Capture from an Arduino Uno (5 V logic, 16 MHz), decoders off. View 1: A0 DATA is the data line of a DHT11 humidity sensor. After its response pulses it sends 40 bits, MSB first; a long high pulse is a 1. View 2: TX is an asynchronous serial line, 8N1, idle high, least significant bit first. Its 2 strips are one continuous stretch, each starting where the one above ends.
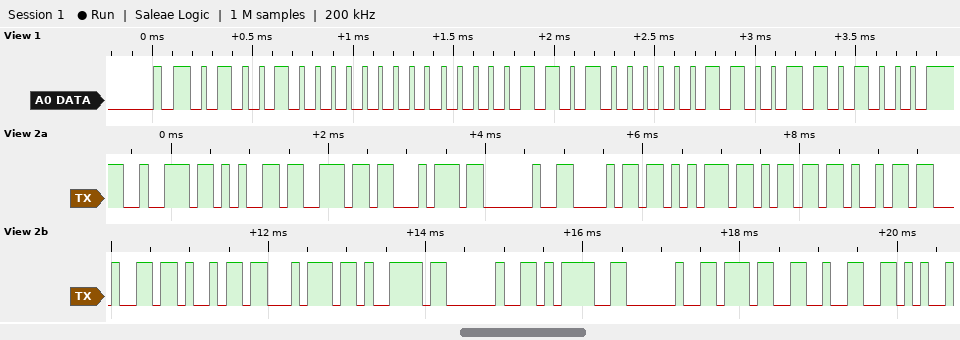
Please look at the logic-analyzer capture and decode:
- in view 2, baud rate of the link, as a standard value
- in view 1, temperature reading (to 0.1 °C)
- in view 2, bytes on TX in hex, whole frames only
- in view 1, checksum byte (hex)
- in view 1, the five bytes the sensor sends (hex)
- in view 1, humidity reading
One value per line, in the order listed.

9600 baud
26.6 °C
72 65 6E 74 20 68 75 6D 69 64 69 74 79 20 3D 20 37 32
0x68
48 00 1A 06 68
72 %
